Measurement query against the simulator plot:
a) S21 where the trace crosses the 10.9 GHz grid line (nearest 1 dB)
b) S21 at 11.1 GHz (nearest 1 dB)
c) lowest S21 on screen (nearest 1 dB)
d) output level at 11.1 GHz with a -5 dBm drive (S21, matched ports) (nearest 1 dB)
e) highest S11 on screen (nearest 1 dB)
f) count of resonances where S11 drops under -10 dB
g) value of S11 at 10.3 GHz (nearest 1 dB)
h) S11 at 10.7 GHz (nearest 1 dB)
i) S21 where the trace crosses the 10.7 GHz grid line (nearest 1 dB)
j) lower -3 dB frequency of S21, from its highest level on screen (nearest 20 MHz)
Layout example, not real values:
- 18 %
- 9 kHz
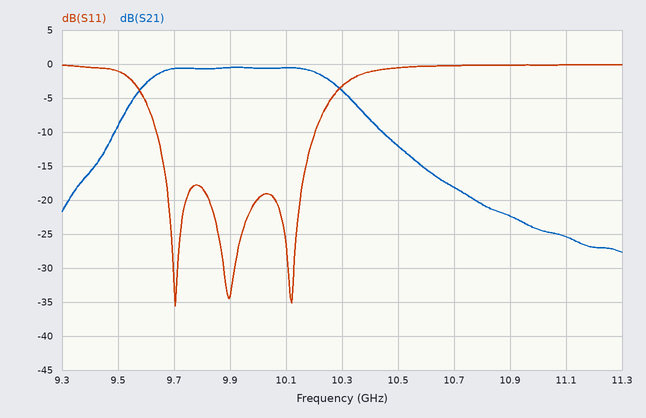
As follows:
- -22 dB
- -25 dB
- -28 dB
- -30 dBm
- 0 dB
- 3
- -3 dB
- 0 dB
- -18 dB
- 9.58 GHz
